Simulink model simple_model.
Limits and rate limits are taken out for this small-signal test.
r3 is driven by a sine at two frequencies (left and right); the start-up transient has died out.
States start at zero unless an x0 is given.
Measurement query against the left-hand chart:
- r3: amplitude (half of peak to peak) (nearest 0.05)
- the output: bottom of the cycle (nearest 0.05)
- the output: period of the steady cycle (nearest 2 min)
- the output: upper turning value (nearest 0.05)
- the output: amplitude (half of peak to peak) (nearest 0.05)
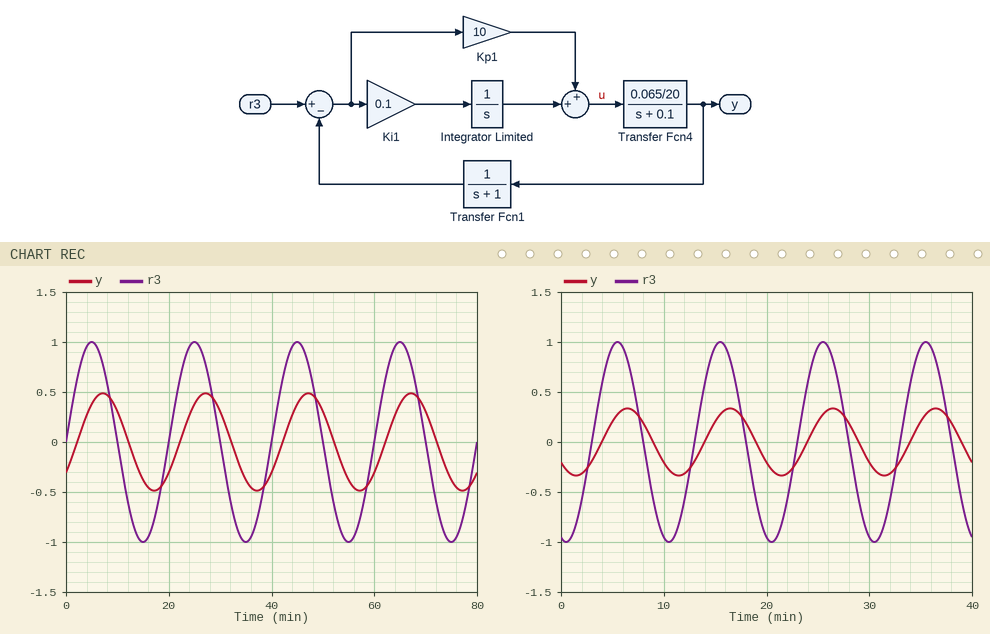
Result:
1.00
-0.50
20 min
0.50
0.50
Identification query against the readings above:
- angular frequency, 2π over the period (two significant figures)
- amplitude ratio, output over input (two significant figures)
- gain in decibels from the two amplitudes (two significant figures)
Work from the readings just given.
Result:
0.31 rad/min
0.50
-6.0 dB
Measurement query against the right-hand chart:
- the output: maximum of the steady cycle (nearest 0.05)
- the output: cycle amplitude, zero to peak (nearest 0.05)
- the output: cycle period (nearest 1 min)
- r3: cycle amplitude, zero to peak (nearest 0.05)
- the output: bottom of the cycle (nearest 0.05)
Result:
0.35
0.35
10 min
1.00
-0.35
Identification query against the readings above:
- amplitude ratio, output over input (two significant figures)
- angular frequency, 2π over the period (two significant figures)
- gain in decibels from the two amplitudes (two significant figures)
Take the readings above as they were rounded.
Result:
0.35
0.63 rad/min
-9.1 dB
